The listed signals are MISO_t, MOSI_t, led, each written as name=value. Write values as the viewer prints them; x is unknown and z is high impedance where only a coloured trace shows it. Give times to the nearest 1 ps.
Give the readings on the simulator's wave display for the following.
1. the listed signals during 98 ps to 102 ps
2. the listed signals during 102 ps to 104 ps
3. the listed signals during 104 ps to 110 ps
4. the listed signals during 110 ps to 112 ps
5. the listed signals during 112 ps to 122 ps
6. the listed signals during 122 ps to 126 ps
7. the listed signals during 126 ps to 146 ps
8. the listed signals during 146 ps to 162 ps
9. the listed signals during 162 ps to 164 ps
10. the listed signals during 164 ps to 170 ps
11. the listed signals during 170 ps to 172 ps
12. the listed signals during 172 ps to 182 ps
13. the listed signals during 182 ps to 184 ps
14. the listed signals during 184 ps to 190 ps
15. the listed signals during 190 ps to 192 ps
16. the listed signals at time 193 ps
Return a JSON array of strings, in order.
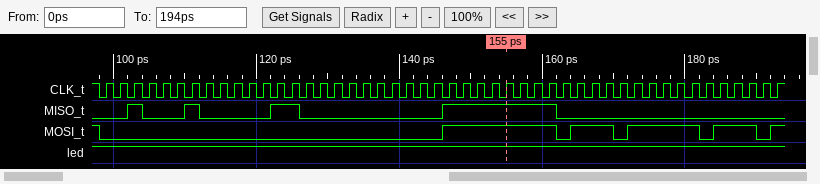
["MISO_t=0, MOSI_t=0, led=1", "MISO_t=1, MOSI_t=0, led=1", "MISO_t=0, MOSI_t=0, led=1", "MISO_t=1, MOSI_t=0, led=1", "MISO_t=0, MOSI_t=0, led=1", "MISO_t=1, MOSI_t=0, led=1", "MISO_t=0, MOSI_t=0, led=1", "MISO_t=1, MOSI_t=1, led=1", "MISO_t=0, MOSI_t=0, led=1", "MISO_t=0, MOSI_t=1, led=1", "MISO_t=0, MOSI_t=0, led=1", "MISO_t=0, MOSI_t=1, led=1", "MISO_t=0, MOSI_t=0, led=1", "MISO_t=0, MOSI_t=1, led=1", "MISO_t=0, MOSI_t=0, led=1", "MISO_t=0, MOSI_t=1, led=1"]
